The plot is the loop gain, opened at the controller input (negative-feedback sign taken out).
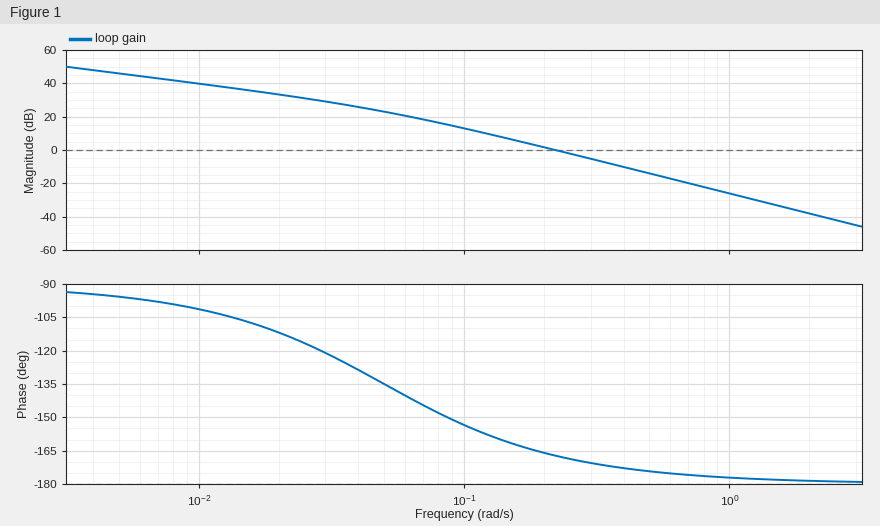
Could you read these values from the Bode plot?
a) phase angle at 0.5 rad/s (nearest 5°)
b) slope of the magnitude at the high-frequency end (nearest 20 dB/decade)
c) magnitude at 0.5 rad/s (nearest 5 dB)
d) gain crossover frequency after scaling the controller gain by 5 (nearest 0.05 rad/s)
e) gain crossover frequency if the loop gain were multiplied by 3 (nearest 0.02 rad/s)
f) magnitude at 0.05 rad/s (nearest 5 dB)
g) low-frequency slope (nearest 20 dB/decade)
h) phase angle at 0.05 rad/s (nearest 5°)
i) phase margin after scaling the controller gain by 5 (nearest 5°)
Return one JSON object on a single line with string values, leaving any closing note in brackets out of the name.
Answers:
{"phase angle at 0.5 rad/s": "-175°", "slope of the magnitude at the high-frequency end": "-40 dB/decade", "magnitude at 0.5 rad/s": "-15 dB", "gain crossover frequency after scaling the controller gain by 5": "0.50 rad/s", "gain crossover frequency if the loop gain were multiplied by 3": "0.38 rad/s", "magnitude at 0.05 rad/s": "25 dB", "low-frequency slope": "-20 dB/decade", "phase angle at 0.05 rad/s": "-135°", "phase margin after scaling the controller gain by 5": "5°"}
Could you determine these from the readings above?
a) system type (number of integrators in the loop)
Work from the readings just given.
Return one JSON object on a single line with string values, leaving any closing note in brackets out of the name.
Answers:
{"system type": "1"}
